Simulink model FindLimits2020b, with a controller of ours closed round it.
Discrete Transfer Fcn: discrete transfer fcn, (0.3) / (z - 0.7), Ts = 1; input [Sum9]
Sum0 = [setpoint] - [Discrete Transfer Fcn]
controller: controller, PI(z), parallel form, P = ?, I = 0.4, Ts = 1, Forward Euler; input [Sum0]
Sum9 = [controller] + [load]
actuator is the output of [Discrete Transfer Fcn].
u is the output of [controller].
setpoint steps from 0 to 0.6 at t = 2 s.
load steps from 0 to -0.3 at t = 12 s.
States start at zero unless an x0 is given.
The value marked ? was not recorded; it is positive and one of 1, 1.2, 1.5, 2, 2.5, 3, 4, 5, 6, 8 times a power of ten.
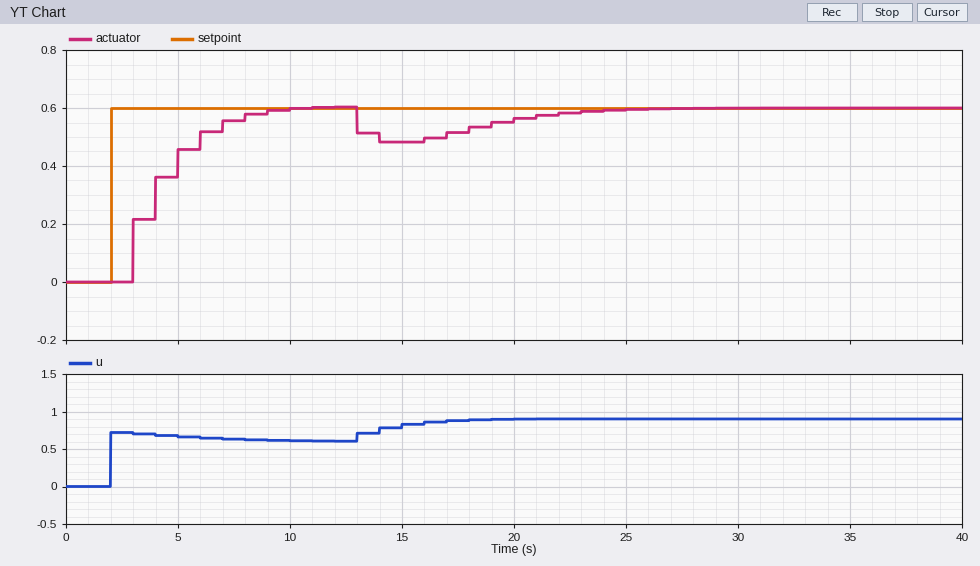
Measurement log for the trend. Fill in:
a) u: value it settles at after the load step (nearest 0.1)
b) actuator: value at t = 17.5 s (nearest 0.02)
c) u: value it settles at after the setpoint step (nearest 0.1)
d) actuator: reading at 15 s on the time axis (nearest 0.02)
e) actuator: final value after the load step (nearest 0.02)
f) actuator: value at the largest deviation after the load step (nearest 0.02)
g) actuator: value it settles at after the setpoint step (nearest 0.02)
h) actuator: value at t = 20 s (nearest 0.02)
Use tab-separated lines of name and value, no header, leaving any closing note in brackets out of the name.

u: value it settles at after the load step	0.9
actuator: value at t = 17.5 s	0.52
u: value it settles at after the setpoint step	0.6
actuator: reading at 15 s on the time axis	0.48
actuator: final value after the load step	0.60
actuator: value at the largest deviation after the load step	0.48
actuator: value it settles at after the setpoint step	0.60
actuator: value at t = 20 s	0.56
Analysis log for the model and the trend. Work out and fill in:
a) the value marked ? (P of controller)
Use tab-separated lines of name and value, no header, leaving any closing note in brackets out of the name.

the value marked ?	1.2
